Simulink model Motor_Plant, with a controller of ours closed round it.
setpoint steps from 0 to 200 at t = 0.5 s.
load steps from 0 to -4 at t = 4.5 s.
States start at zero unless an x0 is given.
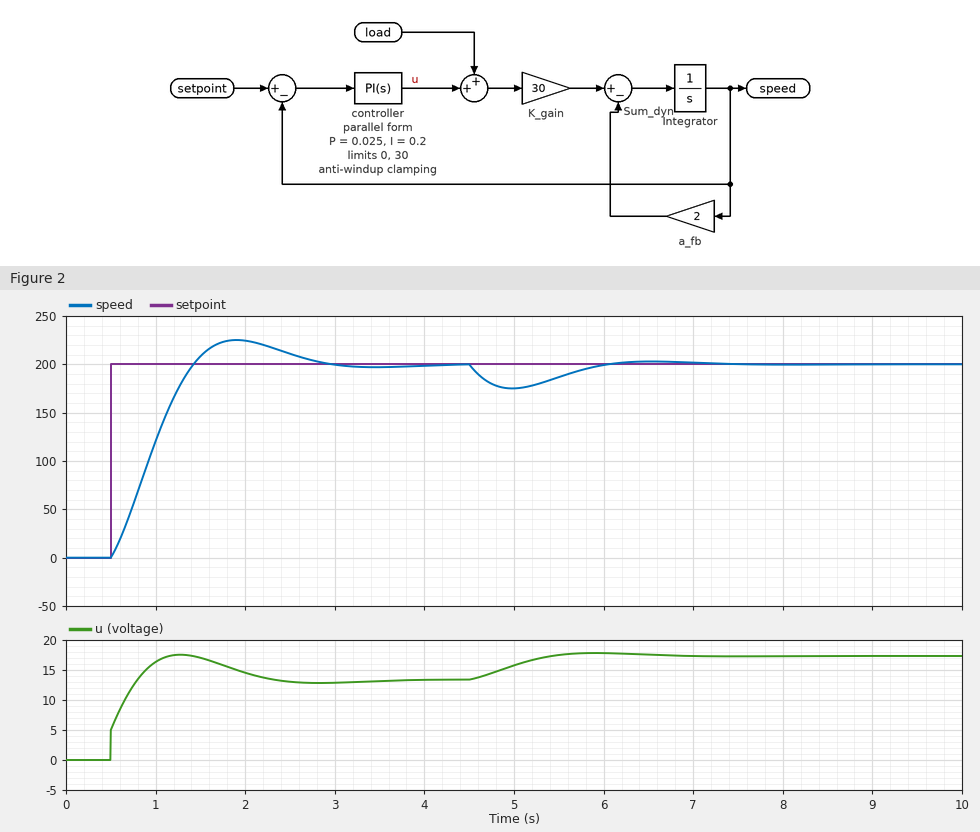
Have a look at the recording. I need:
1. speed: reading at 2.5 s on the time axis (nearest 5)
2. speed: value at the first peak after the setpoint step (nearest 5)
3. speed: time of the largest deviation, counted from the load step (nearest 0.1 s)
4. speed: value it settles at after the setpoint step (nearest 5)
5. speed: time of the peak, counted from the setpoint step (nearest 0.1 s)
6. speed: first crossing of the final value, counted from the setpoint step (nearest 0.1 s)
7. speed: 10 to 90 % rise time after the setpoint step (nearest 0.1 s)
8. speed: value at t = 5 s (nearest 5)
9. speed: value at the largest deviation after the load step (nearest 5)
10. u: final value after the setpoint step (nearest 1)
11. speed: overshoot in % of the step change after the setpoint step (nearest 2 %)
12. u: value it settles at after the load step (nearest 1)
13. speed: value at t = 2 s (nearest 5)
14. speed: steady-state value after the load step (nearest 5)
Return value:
210
225
0.5 s
200
1.4 s
0.9 s
0.7 s
175
175
13
12 %
17
225
200
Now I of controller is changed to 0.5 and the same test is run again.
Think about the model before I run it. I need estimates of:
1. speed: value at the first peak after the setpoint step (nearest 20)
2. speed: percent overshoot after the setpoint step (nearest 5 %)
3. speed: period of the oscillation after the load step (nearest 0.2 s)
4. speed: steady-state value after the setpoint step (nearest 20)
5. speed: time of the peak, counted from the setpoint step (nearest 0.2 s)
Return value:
260
30 %
1.8 s
200
0.8 s
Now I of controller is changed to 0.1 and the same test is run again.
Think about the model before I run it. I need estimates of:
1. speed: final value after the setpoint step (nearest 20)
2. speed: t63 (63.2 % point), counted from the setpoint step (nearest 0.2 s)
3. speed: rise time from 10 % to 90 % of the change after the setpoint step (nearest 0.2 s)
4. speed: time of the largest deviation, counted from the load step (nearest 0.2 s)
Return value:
200
0.8 s
1.2 s
0.6 s
